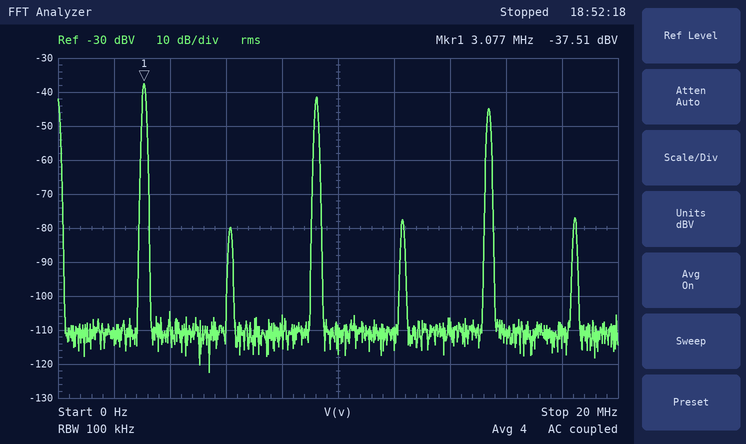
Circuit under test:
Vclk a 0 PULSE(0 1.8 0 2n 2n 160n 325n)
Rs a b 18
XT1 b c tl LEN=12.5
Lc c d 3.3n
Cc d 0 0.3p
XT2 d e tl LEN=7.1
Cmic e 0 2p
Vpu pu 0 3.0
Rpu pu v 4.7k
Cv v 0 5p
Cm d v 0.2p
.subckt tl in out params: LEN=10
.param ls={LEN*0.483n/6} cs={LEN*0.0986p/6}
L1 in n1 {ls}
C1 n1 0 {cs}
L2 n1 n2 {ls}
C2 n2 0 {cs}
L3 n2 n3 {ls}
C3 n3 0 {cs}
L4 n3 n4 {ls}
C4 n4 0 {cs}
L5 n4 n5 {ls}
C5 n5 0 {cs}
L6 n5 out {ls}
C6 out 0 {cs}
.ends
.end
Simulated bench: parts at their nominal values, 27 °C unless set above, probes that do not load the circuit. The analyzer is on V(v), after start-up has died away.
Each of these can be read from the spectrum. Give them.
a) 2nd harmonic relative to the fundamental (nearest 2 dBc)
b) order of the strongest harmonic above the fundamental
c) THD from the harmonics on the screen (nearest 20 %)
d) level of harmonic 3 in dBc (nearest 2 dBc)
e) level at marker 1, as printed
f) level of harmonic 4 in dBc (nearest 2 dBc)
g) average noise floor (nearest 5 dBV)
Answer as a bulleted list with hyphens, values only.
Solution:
- -42 dBc
- 3
- 80 %
- -4 dBc
- -37.51 dBV
- -40 dBc
- -110 dBV
